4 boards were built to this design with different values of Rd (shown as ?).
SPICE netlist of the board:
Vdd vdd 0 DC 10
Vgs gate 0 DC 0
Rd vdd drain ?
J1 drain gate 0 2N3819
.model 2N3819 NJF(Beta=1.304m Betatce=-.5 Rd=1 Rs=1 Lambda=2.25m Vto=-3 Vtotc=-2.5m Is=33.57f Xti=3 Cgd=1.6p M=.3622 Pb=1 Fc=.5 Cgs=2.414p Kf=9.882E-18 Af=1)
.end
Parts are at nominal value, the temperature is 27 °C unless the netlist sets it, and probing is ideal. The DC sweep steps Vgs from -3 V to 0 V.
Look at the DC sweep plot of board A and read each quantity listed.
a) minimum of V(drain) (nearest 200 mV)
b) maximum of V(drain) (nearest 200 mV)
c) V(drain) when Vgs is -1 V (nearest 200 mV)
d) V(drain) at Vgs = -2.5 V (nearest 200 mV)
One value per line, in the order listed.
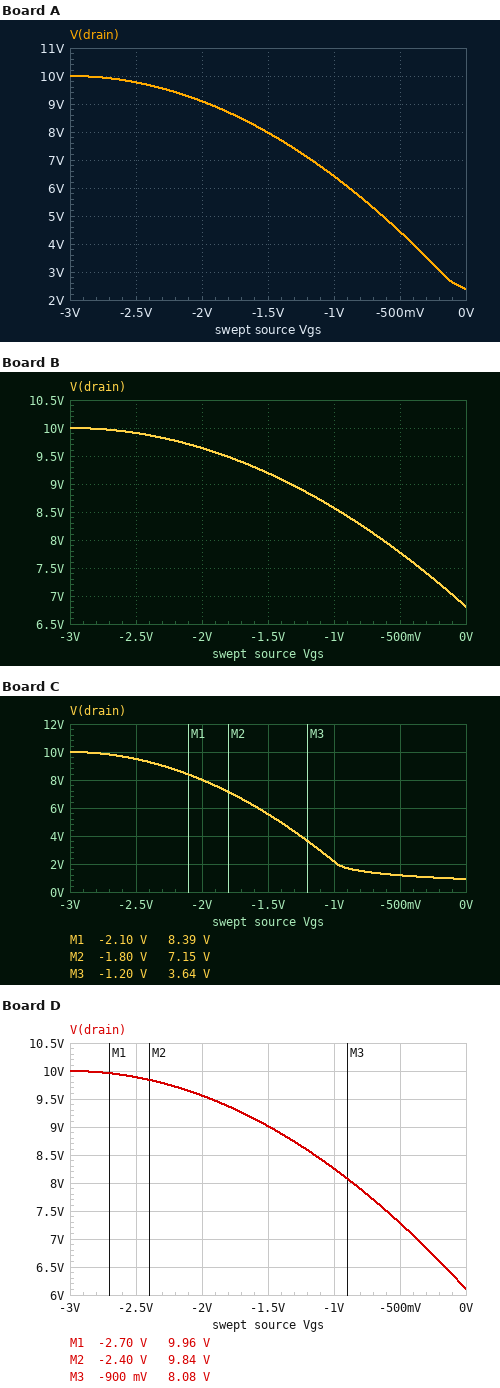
2.4 V
10.0 V
6.4 V
9.8 V
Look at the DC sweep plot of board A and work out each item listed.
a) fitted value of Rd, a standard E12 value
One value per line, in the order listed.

680 Ω
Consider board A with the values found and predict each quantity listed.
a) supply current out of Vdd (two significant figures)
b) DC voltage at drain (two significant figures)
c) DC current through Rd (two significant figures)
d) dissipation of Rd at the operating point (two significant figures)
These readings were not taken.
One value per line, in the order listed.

11 mA
2.4 V
11 mA
85 mW
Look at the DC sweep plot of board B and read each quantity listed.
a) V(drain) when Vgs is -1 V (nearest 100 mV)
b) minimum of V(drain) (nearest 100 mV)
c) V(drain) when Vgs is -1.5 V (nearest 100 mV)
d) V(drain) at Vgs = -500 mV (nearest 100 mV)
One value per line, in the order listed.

8.6 V
6.8 V
9.2 V
7.8 V
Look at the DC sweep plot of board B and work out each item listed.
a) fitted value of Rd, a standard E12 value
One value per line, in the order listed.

270 Ω
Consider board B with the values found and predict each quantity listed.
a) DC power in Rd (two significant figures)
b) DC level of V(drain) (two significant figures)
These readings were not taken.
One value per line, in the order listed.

38 mW
6.8 V
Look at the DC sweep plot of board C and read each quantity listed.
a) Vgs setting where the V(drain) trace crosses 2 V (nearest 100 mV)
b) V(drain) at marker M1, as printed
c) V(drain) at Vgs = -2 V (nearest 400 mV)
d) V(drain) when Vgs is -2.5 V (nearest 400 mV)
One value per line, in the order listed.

-1.0 V
8.39 V
8.0 V
9.6 V
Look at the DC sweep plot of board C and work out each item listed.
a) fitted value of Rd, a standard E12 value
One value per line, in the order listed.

1.5 kΩ
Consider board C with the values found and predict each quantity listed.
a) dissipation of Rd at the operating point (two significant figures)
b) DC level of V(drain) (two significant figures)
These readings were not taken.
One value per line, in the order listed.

55 mW
920 mV
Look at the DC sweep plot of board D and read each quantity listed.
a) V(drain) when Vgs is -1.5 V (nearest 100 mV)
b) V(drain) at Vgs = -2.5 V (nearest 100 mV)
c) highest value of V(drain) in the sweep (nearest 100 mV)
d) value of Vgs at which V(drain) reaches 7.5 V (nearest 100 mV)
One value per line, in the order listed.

9.0 V
9.9 V
10.0 V
-600 mV
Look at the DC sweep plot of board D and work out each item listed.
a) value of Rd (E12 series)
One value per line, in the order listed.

330 Ω
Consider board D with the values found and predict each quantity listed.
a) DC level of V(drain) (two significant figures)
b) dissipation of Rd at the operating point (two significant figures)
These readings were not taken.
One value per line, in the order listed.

6.1 V
46 mW
